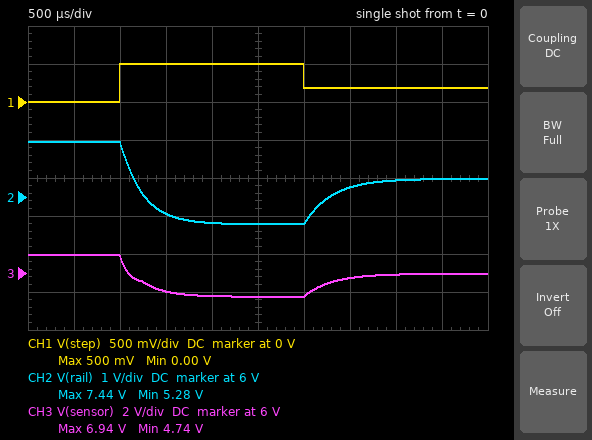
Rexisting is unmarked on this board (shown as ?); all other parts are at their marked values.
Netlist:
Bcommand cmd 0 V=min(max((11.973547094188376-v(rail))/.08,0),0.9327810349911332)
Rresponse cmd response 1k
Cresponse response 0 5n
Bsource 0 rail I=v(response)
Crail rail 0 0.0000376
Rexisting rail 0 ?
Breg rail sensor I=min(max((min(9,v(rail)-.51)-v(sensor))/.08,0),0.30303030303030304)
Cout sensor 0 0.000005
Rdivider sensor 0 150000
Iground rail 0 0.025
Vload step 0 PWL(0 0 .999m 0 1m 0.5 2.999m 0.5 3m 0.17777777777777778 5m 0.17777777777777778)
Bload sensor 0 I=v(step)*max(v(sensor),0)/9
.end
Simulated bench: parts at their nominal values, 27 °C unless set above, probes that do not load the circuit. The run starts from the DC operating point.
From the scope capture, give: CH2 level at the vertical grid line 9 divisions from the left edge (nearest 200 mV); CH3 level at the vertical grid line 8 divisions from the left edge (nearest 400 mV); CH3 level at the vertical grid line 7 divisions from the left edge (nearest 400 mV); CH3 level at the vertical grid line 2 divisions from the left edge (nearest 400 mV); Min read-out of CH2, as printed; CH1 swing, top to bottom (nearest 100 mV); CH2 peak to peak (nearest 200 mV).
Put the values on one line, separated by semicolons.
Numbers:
6.4 V; 6.0 V; 5.6 V; 6.8 V; 5.28 V; 500 mV; 2.2 V
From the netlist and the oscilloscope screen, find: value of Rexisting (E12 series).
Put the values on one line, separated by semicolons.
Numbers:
8.2 Ω
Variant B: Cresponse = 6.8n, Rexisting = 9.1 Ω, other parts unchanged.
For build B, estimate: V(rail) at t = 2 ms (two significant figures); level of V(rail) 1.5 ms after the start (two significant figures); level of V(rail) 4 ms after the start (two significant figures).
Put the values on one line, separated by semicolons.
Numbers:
5.7 V; 6.1 V; 7.0 V
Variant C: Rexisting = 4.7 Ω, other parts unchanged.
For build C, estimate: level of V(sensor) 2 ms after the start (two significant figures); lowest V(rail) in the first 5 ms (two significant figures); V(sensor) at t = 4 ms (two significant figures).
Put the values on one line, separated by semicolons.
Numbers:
3.0 V; 3.5 V; 3.4 V
